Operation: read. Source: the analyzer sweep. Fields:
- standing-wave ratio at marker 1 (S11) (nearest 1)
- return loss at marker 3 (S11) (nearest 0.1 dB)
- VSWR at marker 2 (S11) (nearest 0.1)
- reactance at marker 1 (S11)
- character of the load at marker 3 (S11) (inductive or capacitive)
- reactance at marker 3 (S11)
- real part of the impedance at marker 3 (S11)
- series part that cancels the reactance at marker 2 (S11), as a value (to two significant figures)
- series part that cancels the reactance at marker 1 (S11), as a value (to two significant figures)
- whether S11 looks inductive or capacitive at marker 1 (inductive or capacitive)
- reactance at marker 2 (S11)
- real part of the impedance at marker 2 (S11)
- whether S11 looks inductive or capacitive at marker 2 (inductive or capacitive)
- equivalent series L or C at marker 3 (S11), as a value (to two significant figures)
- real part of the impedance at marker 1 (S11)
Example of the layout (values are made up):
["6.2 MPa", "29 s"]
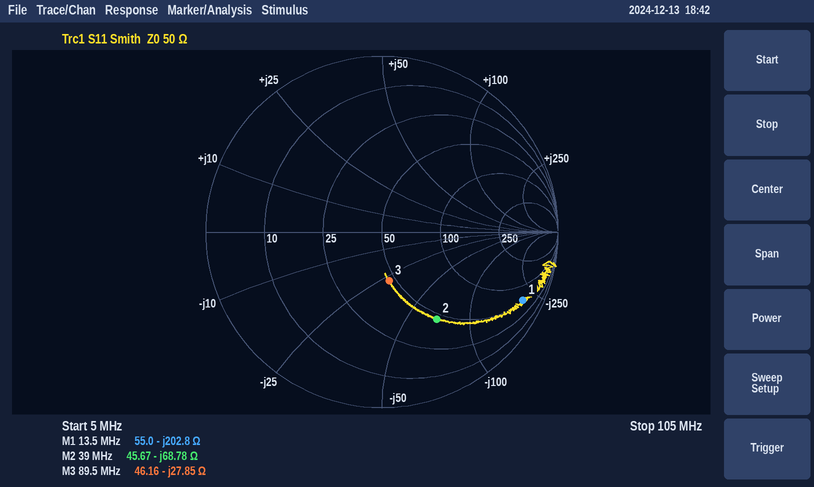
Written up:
["17", "11.0 dB", "3.8", "-202.8 Ω", "capacitive", "-27.85 Ω", "46.16 Ω", "280 nH", "2.4 µH", "capacitive", "-68.78 Ω", "45.67 Ω", "capacitive", "64 pF", "55.0 Ω"]
